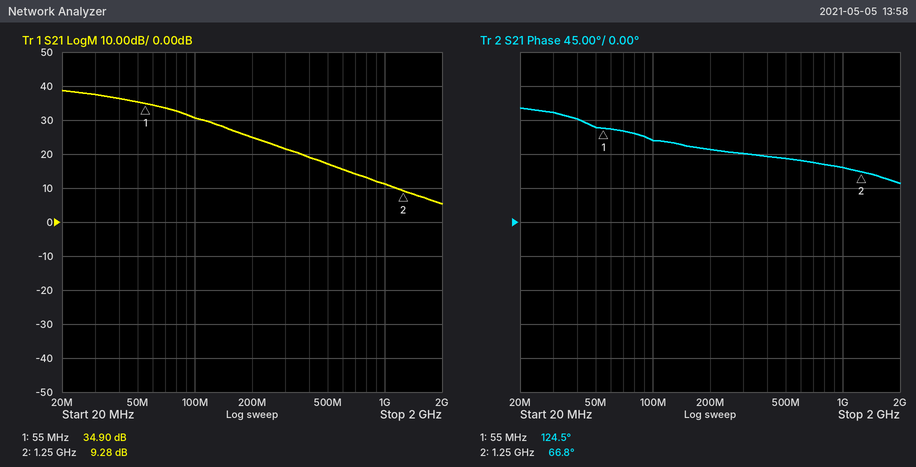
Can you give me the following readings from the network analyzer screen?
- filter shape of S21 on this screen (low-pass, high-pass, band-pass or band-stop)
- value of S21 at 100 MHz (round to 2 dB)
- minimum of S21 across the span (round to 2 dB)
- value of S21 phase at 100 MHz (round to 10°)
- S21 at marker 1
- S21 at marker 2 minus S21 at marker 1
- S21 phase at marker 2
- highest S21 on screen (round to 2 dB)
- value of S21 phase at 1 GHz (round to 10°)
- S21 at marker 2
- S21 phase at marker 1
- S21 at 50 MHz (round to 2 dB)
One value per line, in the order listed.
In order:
low-pass
30 dB
6 dB
110°
34.90 dB
-25.62 dB
66.8°
38 dB
70°
9.28 dB
124.5°
36 dB
